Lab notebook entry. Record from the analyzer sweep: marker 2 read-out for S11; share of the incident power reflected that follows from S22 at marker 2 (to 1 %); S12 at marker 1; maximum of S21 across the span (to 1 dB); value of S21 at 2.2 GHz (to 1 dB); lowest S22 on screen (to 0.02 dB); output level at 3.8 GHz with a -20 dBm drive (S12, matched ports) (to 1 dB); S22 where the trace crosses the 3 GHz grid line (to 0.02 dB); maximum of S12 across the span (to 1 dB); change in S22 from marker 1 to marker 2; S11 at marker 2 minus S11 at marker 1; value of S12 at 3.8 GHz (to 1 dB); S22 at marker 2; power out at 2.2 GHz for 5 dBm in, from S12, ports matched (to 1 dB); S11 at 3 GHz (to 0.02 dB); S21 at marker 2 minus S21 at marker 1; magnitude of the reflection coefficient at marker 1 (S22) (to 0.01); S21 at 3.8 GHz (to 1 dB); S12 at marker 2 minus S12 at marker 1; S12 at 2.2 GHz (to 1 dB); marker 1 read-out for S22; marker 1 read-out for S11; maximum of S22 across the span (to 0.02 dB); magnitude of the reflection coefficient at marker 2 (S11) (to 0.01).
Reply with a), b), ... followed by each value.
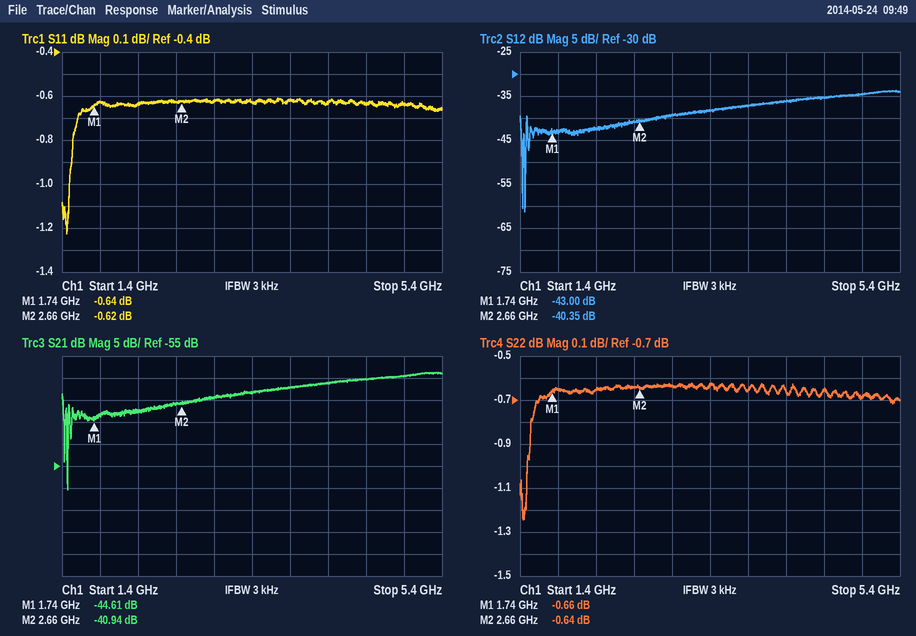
a) -0.62 dB
b) 86 %
c) -43.00 dB
d) -34 dB
e) -42 dB
f) -1.24 dB
g) -57 dBm
h) -0.64 dB
i) -34 dB
j) 0.02 dB
k) 0.02 dB
l) -37 dB
m) -0.64 dB
n) -37 dBm
o) -0.62 dB
p) 3.67 dB
q) 0.93
r) -37 dB
s) 2.65 dB
t) -42 dB
u) -0.66 dB
v) -0.64 dB
w) -0.62 dB
x) 0.93
